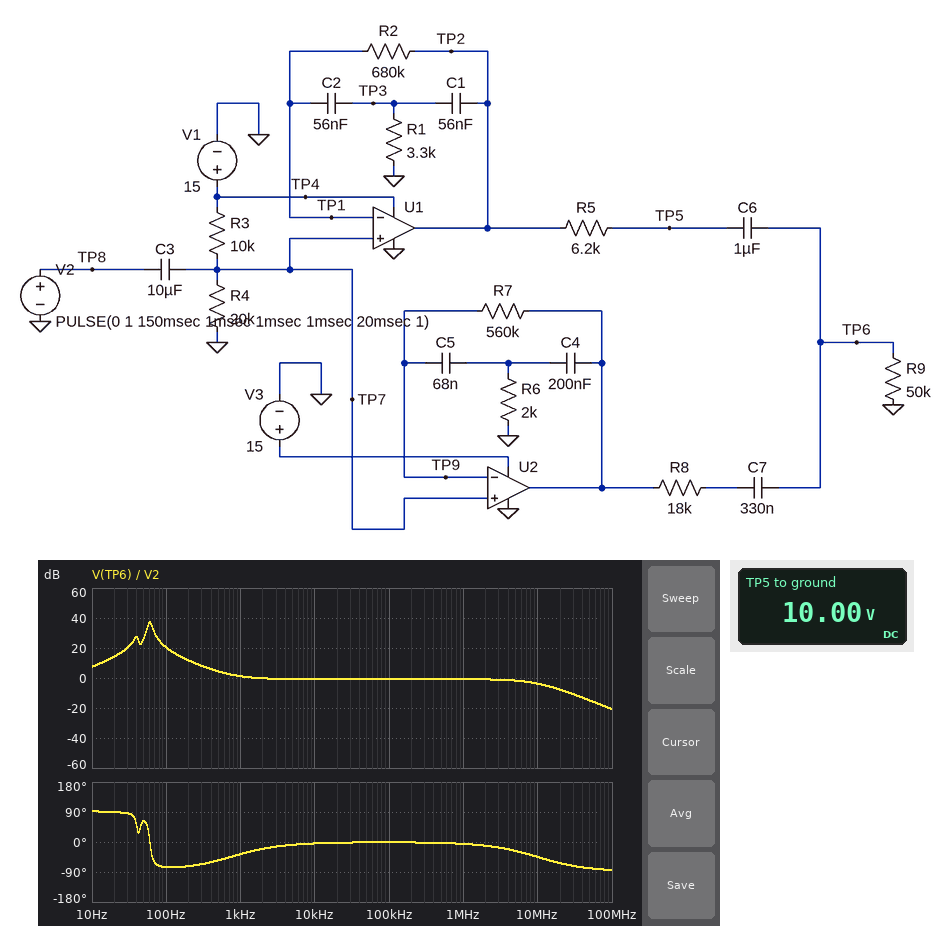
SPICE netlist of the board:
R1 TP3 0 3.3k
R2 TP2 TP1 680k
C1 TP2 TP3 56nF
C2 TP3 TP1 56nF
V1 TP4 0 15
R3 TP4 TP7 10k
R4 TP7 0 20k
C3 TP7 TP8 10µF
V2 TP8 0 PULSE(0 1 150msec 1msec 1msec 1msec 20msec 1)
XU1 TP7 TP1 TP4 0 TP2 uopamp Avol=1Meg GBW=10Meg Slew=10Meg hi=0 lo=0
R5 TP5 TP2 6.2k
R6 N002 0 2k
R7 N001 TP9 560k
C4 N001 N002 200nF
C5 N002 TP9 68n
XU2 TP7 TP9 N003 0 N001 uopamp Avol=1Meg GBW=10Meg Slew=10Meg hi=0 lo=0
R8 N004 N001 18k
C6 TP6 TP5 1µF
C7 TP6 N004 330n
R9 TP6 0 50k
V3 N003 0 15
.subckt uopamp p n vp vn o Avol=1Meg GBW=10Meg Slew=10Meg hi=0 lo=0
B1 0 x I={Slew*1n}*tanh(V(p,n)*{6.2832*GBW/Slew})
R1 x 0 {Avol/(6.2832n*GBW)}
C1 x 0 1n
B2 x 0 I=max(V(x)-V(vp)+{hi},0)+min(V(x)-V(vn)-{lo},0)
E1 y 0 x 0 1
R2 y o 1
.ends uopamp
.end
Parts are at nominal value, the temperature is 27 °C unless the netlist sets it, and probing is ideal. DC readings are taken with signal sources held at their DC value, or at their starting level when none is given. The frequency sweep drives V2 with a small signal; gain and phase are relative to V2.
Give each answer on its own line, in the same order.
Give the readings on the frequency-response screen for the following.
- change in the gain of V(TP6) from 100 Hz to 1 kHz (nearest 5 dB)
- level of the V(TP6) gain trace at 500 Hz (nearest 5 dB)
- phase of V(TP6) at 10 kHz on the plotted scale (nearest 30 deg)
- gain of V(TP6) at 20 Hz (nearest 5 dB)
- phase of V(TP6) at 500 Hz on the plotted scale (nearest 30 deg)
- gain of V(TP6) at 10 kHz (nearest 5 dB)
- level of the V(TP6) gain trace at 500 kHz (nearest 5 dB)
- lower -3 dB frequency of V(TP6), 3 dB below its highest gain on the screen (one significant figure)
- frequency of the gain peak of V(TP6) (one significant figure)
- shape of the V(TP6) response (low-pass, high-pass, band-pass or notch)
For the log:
-20 dB
5 dB
0 deg
15 dB
-60 deg
0 dB
0 dB
60 Hz
60 Hz
band-pass
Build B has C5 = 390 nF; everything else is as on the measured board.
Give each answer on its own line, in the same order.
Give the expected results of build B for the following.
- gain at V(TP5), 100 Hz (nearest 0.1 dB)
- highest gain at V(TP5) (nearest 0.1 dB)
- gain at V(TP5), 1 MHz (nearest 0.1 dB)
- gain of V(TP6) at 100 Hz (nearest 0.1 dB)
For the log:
20.3 dB
37.7 dB
-0.8 dB
20.2 dB
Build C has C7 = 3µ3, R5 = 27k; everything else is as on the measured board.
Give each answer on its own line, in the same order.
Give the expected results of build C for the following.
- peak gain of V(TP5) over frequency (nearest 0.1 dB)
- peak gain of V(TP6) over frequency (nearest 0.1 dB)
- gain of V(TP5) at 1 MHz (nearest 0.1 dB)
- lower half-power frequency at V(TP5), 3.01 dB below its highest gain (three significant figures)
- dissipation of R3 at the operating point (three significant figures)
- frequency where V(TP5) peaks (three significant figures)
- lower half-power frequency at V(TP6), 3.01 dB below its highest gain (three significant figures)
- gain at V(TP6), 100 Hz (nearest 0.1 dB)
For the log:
31.9 dB
31.4 dB
-1.7 dB
37.6 Hz
2.50 mW
40.5 Hz
37.4 Hz
16.7 dB
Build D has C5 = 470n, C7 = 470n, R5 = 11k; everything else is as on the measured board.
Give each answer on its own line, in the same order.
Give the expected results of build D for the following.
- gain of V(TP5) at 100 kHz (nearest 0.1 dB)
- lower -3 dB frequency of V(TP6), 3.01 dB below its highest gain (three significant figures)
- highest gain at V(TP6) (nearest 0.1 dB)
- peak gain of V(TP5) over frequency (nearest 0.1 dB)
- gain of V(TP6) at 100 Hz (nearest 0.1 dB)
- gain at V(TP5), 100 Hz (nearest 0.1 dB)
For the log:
-1.1 dB
14.5 Hz
35.6 dB
35.8 dB
18.9 dB
19.0 dB
